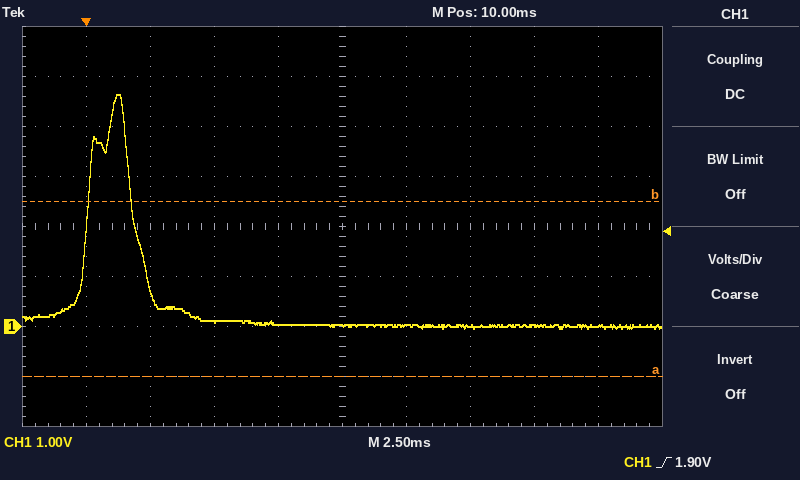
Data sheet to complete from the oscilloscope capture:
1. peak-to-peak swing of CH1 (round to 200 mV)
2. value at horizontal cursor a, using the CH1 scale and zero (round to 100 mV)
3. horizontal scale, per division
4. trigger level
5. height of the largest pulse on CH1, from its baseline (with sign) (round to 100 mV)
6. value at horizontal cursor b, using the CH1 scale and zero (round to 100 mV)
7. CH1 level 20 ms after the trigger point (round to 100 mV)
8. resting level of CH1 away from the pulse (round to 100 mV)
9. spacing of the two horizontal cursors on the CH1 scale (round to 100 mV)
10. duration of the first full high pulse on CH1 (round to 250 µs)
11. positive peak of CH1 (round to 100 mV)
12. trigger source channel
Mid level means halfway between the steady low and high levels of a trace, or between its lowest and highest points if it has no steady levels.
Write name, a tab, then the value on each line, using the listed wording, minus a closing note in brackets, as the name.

peak-to-peak swing of CH1	4.6 V
value at horizontal cursor a, using the CH1 scale and zero	-1.0 V
horizontal scale, per division	2.5 ms
trigger level	1.90 V
height of the largest pulse on CH1, from its baseline (with sign)	+4.6 V
value at horizontal cursor b, using the CH1 scale and zero	2.5 V
CH1 level 20 ms after the trigger point	0.0 V
resting level of CH1 away from the pulse	0.0 V
spacing of the two horizontal cursors on the CH1 scale	3.5 V
duration of the first full high pulse on CH1	1.75 ms
positive peak of CH1	4.6 V
trigger source channel	CH1
